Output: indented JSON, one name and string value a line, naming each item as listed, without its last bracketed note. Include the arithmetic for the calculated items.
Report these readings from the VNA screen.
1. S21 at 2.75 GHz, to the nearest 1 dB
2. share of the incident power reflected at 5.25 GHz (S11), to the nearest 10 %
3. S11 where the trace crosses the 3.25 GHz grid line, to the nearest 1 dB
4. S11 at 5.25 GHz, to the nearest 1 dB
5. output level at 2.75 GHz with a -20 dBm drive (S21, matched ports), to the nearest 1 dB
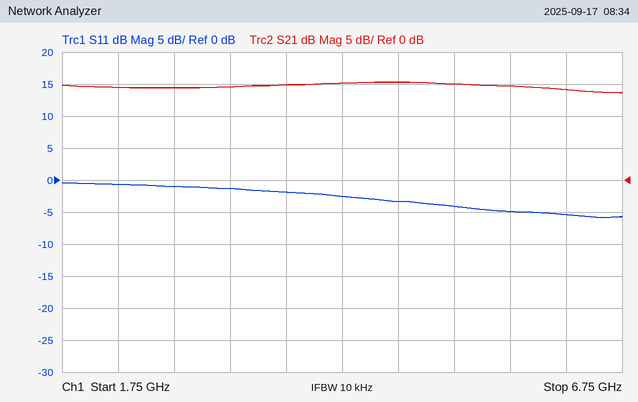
{
  "S21 at 2.75 GHz, to the nearest 1 dB": "14 dB",
  "share of the incident power reflected at 5.25 GHz (S11), to the nearest 10 %": "10^(-4/10) ≈ 40 %",
  "S11 where the trace crosses the 3.25 GHz grid line, to the nearest 1 dB": "-1 dB",
  "S11 at 5.25 GHz, to the nearest 1 dB": "-4 dB",
  "output level at 2.75 GHz with a -20 dBm drive (S21, matched ports), to the nearest 1 dB": "-20 dBm + (14 dB) = -6 dBm"
}
